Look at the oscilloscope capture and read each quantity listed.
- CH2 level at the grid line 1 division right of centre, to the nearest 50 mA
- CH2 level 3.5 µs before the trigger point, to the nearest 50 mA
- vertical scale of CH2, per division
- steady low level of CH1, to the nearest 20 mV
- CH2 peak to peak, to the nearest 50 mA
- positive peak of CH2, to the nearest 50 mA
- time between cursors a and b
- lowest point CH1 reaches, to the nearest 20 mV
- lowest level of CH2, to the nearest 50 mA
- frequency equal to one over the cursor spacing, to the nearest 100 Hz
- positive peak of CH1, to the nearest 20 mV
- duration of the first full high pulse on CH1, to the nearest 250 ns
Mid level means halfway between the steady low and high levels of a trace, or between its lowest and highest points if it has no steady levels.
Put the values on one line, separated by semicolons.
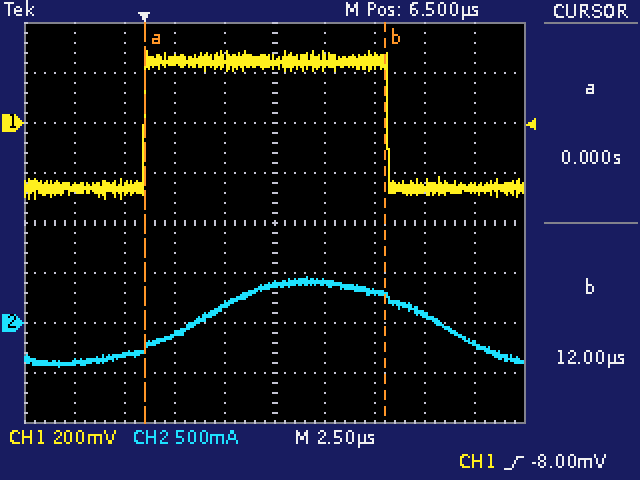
400 mA; -400 mA; 500 mA; -260 mV; 900 mA; 450 mA; 12.00 µs; -300 mV; -450 mA; 83.3 kHz; 280 mV; 12.25 µs
